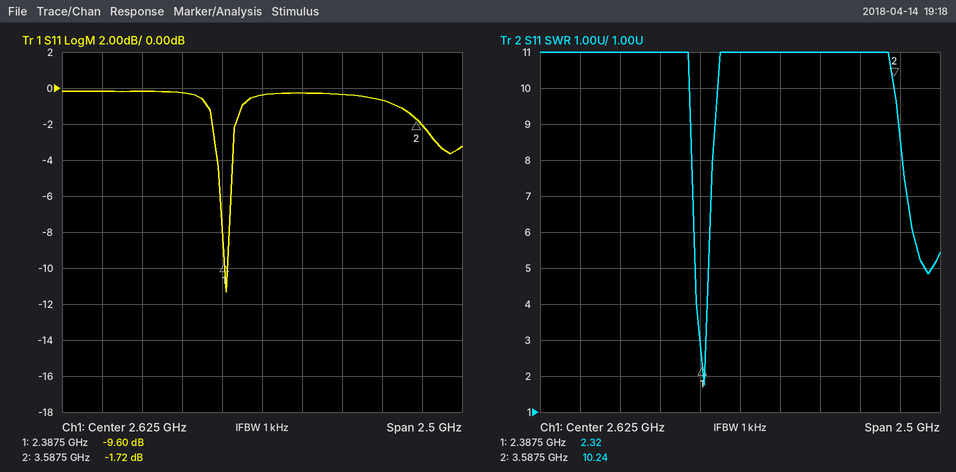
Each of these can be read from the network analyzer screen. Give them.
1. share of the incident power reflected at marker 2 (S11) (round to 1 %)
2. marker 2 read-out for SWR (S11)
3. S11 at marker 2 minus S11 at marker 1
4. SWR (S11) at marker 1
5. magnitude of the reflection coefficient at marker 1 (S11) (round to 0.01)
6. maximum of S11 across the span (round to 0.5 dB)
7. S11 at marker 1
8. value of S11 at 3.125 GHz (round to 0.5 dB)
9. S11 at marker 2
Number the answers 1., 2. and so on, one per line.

1. 67 %
2. 10.24
3. 7.88 dB
4. 2.32
5. 0.33
6. 0.0 dB
7. -9.60 dB
8. -0.5 dB
9. -1.72 dB
